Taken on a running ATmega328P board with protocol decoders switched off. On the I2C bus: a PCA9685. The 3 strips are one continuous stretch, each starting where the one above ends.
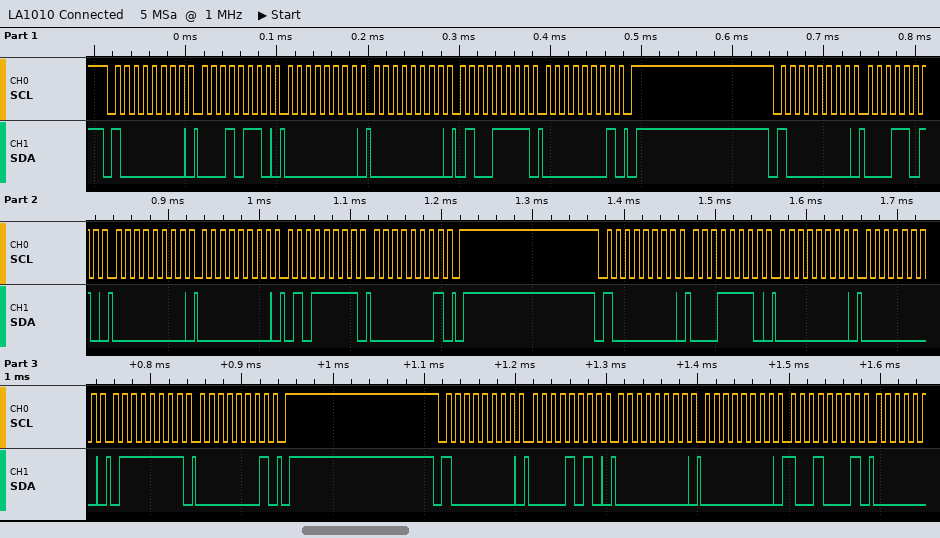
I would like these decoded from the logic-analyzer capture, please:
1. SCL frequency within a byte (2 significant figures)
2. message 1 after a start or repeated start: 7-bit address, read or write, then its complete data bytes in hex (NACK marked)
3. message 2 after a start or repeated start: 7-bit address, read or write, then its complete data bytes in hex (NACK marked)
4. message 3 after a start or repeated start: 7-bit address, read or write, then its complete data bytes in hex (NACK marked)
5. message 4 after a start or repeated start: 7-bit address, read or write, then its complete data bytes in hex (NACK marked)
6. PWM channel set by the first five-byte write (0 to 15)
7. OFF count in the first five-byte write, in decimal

100 kHz
0x40 write: 16 00 00 4F 01
0x40 write: 1A 00 00 5F 01
0x40 write: 1E 00 00 7F 01
0x40 write: 0A 00 00 91
4
335
